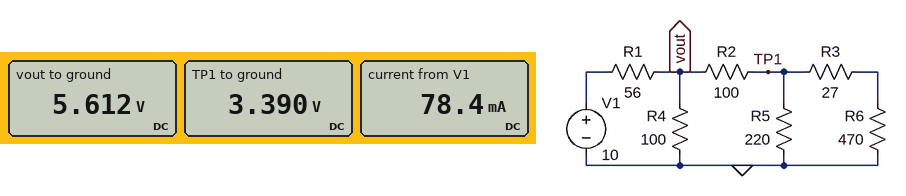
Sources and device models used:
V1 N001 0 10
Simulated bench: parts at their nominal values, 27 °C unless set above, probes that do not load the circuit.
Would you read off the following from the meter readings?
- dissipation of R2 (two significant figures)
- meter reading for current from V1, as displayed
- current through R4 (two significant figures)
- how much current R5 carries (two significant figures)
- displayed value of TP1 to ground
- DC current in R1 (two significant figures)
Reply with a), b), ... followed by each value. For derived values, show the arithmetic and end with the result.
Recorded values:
a) (5.612 V - 3.39 V)^2 / 100 Ω = 49 mW
b) 78.4 mA
c) (5.612 V) / 100 Ω = 56 mA
d) (3.39 V) / 220 Ω = 15 mA
e) 3.390 V
f) (10 V - 5.612 V) / 56 Ω = 78 mA
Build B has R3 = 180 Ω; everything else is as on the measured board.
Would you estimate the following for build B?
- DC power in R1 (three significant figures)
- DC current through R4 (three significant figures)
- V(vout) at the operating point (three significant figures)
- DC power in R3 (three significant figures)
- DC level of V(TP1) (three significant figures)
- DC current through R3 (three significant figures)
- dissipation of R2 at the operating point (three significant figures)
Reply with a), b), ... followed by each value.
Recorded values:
a) 339 mW
b) 56.4 mA
c) 5.64 V
d) 5.25 mW
e) 3.51 V
f) 5.40 mA
g) 45.6 mW
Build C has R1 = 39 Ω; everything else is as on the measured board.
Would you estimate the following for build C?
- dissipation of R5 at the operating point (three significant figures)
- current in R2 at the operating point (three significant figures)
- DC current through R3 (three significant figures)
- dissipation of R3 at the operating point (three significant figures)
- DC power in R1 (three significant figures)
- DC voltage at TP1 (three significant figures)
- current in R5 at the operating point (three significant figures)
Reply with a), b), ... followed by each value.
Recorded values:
a) 69.5 mW
b) 25.6 mA
c) 7.87 mA
d) 1.67 mW
e) 319 mW
f) 3.91 V
g) 17.8 mA
